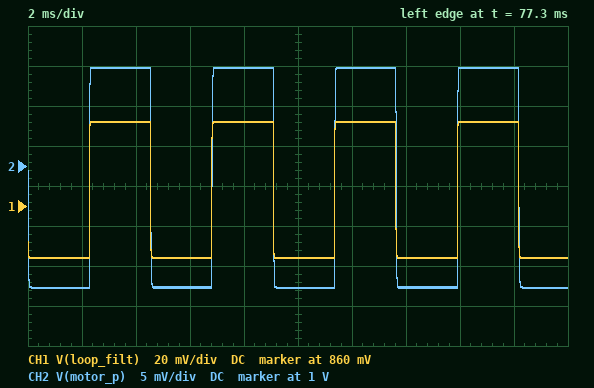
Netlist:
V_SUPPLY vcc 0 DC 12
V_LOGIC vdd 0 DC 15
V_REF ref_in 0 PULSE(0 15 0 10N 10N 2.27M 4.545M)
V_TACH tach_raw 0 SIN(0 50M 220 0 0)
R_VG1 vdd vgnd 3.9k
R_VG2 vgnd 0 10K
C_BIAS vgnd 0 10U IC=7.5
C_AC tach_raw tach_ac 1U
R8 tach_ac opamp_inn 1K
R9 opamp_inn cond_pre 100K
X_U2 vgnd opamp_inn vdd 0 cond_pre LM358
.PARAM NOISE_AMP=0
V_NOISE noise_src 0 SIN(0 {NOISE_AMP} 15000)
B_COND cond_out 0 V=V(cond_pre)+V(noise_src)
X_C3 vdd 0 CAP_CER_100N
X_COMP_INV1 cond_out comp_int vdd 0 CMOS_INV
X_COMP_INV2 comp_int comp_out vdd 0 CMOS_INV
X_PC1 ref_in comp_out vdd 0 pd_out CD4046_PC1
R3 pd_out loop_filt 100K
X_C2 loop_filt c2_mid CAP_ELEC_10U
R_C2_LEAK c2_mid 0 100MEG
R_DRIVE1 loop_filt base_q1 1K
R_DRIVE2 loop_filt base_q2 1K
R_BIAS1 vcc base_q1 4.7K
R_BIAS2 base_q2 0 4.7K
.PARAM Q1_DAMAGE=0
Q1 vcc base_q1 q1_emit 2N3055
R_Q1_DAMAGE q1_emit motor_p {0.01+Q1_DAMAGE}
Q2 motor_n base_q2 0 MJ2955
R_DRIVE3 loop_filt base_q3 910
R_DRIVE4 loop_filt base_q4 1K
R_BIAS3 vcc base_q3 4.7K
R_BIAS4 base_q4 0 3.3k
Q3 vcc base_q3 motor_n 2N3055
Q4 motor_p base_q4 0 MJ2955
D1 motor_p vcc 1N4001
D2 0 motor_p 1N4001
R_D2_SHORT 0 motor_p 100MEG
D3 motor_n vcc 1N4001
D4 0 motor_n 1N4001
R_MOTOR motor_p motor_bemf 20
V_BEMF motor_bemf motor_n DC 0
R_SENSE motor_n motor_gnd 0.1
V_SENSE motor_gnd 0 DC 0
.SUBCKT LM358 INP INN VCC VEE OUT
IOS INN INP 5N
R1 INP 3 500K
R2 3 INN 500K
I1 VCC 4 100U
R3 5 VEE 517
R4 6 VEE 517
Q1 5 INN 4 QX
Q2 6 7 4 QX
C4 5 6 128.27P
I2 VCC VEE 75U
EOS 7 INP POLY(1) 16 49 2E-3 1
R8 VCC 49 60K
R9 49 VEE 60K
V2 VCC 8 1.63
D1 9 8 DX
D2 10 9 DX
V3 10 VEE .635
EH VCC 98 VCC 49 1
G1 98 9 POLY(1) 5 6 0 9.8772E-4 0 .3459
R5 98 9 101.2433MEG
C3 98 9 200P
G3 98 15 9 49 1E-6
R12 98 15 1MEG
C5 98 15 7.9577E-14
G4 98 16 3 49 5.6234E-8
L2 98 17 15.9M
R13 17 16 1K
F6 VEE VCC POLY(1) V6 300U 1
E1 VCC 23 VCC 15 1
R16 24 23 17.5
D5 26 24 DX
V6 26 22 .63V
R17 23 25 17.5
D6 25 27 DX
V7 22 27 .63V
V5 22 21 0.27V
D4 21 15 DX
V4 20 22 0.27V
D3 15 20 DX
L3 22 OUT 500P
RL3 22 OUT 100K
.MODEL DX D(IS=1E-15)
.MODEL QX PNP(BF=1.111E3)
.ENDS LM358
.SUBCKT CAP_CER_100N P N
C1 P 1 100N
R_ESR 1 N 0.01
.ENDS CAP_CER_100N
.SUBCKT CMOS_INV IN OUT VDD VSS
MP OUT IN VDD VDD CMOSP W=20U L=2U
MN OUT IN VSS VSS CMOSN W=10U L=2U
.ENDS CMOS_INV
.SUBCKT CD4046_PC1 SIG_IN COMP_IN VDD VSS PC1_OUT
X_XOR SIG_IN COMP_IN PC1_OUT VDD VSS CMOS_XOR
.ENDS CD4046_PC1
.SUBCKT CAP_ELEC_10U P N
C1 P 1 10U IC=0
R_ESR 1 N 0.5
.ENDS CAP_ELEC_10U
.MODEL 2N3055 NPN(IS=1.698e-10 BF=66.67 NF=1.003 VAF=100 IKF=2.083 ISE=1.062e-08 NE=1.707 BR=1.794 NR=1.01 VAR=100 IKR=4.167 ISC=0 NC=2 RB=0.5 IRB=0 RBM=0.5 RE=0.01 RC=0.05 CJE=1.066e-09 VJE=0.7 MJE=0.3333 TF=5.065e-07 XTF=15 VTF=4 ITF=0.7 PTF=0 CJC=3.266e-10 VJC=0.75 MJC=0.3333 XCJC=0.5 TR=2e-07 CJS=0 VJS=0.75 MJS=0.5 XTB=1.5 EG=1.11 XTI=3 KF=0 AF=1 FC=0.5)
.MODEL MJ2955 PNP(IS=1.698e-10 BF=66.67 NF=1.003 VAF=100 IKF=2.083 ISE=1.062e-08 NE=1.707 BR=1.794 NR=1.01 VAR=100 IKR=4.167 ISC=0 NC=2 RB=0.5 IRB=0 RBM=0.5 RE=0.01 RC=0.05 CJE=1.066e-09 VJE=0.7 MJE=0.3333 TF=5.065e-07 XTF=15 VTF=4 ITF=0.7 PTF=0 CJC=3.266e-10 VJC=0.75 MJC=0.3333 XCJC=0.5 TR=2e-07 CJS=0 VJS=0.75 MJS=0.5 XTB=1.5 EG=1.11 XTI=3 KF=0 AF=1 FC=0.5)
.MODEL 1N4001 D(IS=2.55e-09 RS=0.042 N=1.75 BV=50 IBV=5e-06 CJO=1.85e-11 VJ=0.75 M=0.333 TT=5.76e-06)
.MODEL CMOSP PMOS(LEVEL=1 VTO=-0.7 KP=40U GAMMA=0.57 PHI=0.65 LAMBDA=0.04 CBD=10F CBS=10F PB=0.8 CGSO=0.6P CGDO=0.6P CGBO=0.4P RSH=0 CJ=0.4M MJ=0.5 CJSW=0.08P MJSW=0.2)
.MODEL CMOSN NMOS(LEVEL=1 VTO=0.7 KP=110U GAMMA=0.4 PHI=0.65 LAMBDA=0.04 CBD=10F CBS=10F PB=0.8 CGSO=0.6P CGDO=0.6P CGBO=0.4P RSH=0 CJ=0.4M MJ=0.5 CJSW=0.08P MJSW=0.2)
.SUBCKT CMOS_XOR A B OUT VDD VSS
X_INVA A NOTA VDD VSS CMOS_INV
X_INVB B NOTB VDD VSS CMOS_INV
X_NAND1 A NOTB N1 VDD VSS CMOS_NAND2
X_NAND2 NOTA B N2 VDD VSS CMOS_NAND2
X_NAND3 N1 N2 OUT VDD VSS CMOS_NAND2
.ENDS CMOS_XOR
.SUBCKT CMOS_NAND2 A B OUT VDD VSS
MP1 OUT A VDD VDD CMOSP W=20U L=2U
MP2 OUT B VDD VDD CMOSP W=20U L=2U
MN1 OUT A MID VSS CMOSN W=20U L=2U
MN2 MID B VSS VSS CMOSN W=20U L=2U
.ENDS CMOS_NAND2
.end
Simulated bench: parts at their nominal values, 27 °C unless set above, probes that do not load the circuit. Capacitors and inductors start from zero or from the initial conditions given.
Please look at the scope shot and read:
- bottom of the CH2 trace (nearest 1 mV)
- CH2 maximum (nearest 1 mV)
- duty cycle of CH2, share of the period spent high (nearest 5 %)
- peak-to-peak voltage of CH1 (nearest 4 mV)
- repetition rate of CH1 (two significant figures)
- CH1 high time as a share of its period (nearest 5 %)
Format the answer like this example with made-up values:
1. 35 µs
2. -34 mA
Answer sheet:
1. 985 mV
2. 1.012 V
3. 50 %
4. 68 mV
5. 220 Hz
6. 50 %
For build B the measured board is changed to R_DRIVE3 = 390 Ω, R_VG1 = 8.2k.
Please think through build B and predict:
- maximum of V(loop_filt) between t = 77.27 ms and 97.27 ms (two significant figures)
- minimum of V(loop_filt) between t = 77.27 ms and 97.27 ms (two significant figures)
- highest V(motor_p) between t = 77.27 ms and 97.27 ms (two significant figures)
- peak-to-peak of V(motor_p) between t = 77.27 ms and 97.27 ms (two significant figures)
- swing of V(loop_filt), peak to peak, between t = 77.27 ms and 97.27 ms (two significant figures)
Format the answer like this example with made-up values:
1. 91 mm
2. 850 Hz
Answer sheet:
1. 760 mV
2. 720 mV
3. 960 mV
4. 17 mV
5. 41 mV
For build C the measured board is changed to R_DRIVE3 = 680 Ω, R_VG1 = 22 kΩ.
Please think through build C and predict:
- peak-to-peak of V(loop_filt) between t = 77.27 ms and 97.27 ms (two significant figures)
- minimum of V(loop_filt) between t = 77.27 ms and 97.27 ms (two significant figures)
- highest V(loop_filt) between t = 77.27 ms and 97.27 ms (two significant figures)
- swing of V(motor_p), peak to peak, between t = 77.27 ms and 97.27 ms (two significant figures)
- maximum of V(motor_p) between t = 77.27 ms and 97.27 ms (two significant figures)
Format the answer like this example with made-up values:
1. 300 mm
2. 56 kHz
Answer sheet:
1. 58 mV
2. 790 mV
3. 850 mV
4. 23 mV
5. 990 mV
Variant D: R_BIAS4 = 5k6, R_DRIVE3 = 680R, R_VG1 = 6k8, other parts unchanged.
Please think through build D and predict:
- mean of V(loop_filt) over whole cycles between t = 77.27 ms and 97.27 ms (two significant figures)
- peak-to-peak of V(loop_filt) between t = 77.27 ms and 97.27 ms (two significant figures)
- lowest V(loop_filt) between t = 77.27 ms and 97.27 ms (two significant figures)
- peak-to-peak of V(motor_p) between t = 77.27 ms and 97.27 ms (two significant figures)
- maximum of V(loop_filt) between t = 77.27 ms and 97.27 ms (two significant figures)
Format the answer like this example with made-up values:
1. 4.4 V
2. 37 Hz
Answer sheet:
1. 840 mV
2. 62 mV
3. 810 mV
4. 25 mV
5. 870 mV
